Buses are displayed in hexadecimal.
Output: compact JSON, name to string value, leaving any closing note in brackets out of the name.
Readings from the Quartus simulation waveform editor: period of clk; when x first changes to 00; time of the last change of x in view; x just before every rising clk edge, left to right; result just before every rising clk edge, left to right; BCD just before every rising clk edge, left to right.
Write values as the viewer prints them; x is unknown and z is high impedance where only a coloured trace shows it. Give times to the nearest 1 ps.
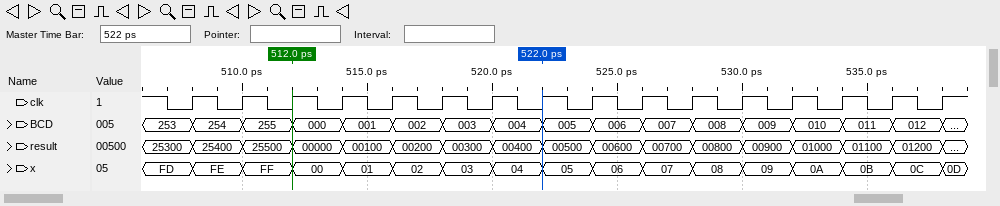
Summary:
{"period of clk": "2 ps", "when x first changes to 00": "512 ps", "time of the last change of x in view": "538 ps", "x just before every rising clk edge, left to right": "FD, FE, FF, 00, 01, 02, 03, 04, 05, 06, 07, 08, 09, 0A, 0B, 0C", "result just before every rising clk edge, left to right": "25300, 25400, 25500, 00000, 00100, 00200, 00300, 00400, 00500, 00600, 00700, 00800, 00900, 01000, 01100, 01200", "BCD just before every rising clk edge, left to right": "253, 254, 255, 000, 001, 002, 003, 004, 005, 006, 007, 008, 009, 010, 011, 012"}
